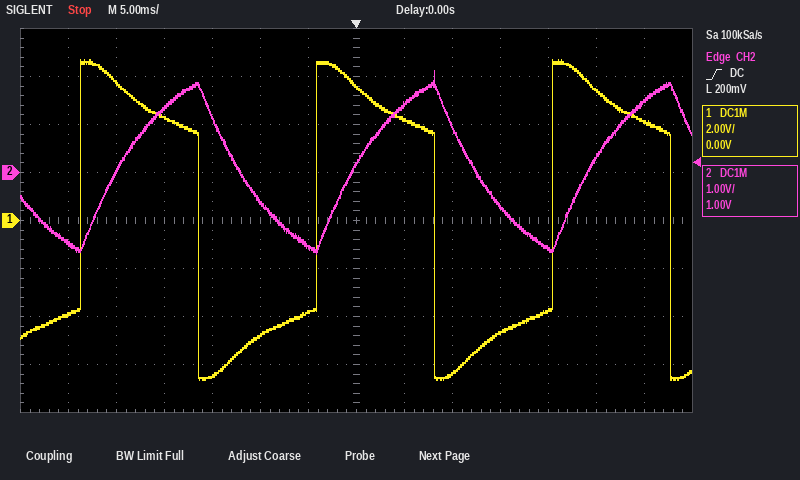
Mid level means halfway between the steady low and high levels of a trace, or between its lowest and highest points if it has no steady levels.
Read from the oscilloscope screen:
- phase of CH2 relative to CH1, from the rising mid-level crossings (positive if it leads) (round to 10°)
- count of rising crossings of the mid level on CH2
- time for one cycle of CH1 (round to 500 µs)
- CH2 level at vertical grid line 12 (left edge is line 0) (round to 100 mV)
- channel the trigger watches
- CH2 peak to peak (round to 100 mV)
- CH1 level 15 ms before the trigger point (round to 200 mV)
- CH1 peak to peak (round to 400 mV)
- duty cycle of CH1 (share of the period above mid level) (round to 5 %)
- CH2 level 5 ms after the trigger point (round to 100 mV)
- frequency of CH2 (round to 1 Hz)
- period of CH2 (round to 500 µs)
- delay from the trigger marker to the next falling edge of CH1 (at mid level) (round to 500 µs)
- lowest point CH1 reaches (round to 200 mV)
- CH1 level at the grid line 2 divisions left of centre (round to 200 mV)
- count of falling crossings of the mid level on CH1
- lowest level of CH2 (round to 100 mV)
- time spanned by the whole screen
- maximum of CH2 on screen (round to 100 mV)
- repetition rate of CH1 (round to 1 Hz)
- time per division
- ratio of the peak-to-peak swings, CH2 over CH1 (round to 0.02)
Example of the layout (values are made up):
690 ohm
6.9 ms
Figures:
-60°
3
24.5 ms
300 mV
CH2
3.8 V
-6.4 V
13.2 V
50 %
1.4 V
41 Hz
24.5 ms
8.0 ms
-6.6 V
-4.8 V
3
-1.7 V
70 ms
2.1 V
41 Hz
5 ms
0.28
